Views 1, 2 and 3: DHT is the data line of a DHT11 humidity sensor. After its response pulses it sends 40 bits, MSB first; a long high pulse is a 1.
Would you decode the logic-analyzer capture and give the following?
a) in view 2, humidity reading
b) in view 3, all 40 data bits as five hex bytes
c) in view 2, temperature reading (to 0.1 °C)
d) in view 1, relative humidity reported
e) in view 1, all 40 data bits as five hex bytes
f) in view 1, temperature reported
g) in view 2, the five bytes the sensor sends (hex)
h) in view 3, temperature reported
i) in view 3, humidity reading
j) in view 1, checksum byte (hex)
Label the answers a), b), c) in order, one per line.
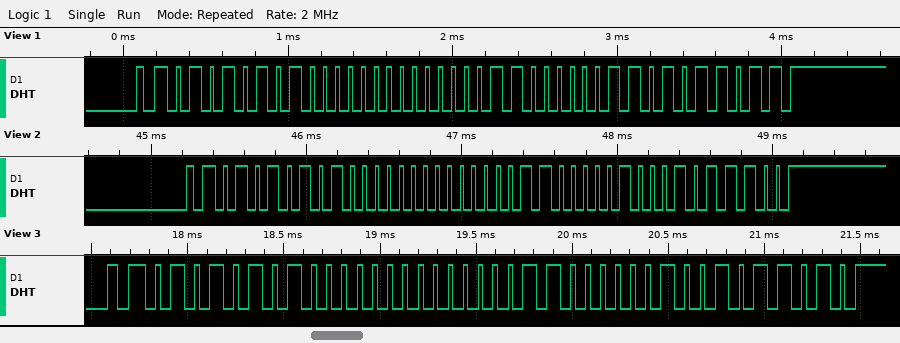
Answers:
a) 85 %
b) 55 00 03 02 5A
c) 3.4 °C
d) 85 %
e) 55 00 03 03 5B
f) 3.3 °C
g) 55 00 03 04 5C
h) 3.2 °C
i) 85 %
j) 0x5B
